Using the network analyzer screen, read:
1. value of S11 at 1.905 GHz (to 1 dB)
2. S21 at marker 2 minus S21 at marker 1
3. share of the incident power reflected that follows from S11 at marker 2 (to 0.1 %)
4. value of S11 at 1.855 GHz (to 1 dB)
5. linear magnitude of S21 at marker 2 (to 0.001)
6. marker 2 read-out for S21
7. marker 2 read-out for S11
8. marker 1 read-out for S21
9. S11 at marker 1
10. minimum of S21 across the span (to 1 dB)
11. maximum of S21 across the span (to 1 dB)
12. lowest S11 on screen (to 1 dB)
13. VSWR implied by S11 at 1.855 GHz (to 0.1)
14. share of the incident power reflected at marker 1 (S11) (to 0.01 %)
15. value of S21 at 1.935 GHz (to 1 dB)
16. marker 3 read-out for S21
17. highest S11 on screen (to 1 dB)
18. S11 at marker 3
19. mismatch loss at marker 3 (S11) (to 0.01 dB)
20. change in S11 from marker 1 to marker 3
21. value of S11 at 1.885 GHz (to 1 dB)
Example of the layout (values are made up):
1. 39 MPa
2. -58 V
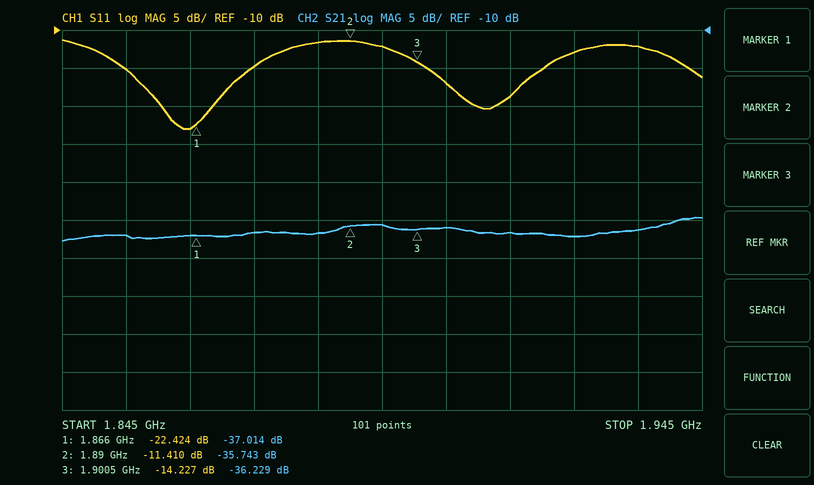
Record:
1. -17 dB
2. 1.271 dB
3. 7.2 %
4. -15 dB
5. 0.016
6. -35.743 dB
7. -11.410 dB
8. -37.014 dB
9. -22.424 dB
10. -38 dB
11. -35 dB
12. -23 dB
13. 1.4
14. 0.57 %
15. -36 dB
16. -36.229 dB
17. -11 dB
18. -14.227 dB
19. 0.17 dB
20. 8.197 dB
21. -12 dB
